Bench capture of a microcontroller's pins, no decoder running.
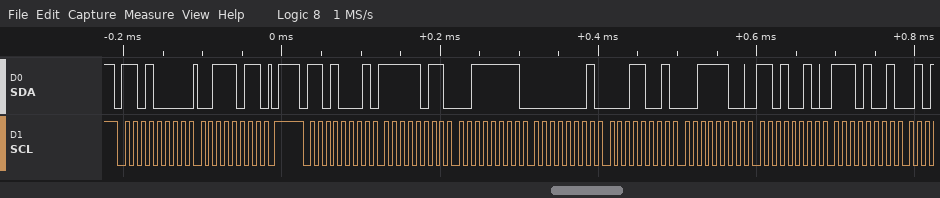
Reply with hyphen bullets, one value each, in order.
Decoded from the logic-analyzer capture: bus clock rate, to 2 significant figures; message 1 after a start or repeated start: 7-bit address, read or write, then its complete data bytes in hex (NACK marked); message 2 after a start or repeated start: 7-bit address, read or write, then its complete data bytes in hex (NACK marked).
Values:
- 100 kHz
- 0x68 write: 3B
- 0x68 read: FB 3F 01 19 3C D2 E9
